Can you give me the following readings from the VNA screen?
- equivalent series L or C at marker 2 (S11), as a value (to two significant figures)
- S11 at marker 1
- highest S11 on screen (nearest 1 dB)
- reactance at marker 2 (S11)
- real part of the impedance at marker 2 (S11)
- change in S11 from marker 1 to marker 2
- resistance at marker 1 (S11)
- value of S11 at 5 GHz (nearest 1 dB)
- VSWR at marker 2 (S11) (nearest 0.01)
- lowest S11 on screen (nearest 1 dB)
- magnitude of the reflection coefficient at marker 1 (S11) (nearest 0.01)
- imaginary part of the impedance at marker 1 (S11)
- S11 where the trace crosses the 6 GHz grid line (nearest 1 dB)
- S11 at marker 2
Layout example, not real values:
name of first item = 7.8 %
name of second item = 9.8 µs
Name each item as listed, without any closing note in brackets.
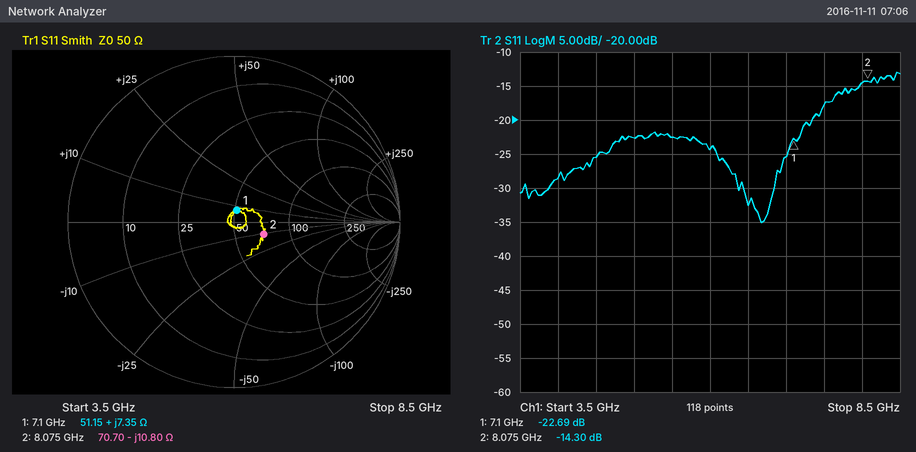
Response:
equivalent series L or C at marker 2 (S11), as a value = 1.8 pF
S11 at marker 1 = -22.69 dB
highest S11 on screen = -13 dB
reactance at marker 2 = -10.80 Ω
real part of the impedance at marker 2 = 70.70 Ω
change in S11 from marker 1 to marker 2 = 8.39 dB
resistance at marker 1 = 51.15 Ω
value of S11 at 5 GHz = -23 dB
VSWR at marker 2 (S11) = 1.48
lowest S11 on screen = -35 dB
magnitude of the reflection coefficient at marker 1 (S11) = 0.07
imaginary part of the impedance at marker 1 = +7.35 Ω
S11 where the trace crosses the 6 GHz grid line = -24 dB
S11 at marker 2 = -14.30 dB
